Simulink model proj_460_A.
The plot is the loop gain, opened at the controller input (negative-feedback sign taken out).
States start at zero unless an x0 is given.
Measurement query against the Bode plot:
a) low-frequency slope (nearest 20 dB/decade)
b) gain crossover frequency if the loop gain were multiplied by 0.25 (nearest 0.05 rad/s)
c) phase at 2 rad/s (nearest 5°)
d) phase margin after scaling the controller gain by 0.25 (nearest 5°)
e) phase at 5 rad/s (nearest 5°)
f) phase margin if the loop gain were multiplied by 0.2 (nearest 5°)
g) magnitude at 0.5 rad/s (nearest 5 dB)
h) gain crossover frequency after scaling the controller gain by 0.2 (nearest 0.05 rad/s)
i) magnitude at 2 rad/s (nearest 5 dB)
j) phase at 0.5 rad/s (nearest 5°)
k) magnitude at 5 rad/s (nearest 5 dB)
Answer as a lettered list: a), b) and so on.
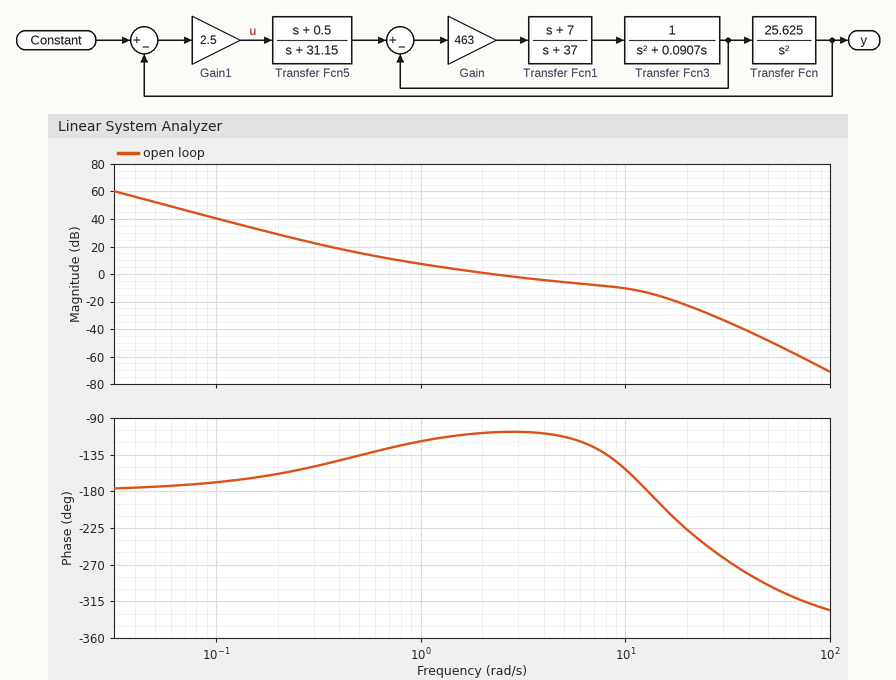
a) -40 dB/decade
b) 0.65 rad/s
c) -110°
d) 50°
e) -115°
f) 45°
g) 15 dB
h) 0.55 rad/s
i) 0 dB
j) -135°
k) -5 dB
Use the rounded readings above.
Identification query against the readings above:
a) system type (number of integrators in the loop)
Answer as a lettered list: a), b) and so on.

a) 2
